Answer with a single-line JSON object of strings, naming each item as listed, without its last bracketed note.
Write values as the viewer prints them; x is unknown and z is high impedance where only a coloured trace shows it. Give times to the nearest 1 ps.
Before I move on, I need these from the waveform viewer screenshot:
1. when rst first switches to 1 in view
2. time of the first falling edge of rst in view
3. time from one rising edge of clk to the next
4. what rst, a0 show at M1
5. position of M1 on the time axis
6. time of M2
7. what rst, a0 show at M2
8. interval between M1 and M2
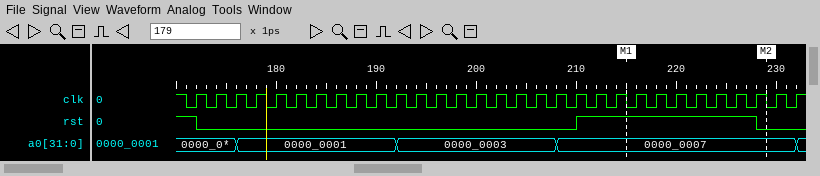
{"when rst first switches to 1 in view": "210 ps", "time of the first falling edge of rst in view": "172 ps", "time from one rising edge of clk to the next": "2 ps", "what rst, a0 show at M1": "rst=1, a0=0000_0007", "position of M1 on the time axis": "215 ps", "time of M2": "229 ps", "what rst, a0 show at M2": "rst=0, a0=0000_0007", "interval between M1 and M2": "14 ps"}
